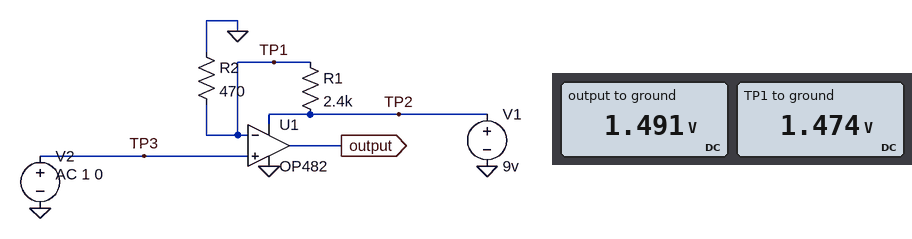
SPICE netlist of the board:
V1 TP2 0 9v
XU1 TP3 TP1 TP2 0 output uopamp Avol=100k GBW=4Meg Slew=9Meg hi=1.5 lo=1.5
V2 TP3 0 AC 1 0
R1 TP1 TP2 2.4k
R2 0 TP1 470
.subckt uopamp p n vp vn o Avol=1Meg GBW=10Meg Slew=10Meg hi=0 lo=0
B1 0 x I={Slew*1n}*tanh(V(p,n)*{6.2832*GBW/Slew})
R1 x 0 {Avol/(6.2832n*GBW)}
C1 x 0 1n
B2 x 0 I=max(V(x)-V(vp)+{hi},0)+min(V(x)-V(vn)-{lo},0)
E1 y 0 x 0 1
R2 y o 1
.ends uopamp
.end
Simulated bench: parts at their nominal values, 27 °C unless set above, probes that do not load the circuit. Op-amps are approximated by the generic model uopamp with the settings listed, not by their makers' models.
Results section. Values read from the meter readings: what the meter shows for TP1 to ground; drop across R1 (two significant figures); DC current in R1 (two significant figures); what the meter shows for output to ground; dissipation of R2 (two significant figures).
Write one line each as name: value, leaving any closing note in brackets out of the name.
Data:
what the meter shows for TP1 to ground: 1.474 V
drop across R1: 7.5 V
DC current in R1: 3.1 mA
what the meter shows for output to ground: 1.491 V
dissipation of R2: 4.6 mW
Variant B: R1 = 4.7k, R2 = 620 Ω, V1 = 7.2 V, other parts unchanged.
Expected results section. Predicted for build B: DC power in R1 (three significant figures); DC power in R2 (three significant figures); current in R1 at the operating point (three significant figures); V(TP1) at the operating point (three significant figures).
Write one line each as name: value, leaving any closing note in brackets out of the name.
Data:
DC power in R1: 8.61 mW
DC power in R2: 1.14 mW
current in R1 at the operating point: 1.35 mA
V(TP1) at the operating point: 839 mV
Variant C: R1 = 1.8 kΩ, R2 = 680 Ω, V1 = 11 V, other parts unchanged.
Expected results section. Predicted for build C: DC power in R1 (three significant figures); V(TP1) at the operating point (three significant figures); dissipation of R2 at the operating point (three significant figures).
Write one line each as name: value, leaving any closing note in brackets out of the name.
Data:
DC power in R1: 35.4 mW
V(TP1) at the operating point: 3.02 V
dissipation of R2 at the operating point: 13.4 mW
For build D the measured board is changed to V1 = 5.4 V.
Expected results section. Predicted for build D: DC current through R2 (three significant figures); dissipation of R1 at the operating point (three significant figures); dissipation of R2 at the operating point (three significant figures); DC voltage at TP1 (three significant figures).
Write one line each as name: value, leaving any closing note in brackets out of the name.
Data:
DC current through R2: 1.88 mA
dissipation of R1 at the operating point: 8.50 mW
dissipation of R2 at the operating point: 1.66 mW
DC voltage at TP1: 884 mV
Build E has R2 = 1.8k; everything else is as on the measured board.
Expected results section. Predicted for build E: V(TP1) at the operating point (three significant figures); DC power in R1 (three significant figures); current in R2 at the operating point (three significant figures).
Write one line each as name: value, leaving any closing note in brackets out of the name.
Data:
V(TP1) at the operating point: 3.86 V
DC power in R1: 11.0 mW
current in R2 at the operating point: 2.14 mA
